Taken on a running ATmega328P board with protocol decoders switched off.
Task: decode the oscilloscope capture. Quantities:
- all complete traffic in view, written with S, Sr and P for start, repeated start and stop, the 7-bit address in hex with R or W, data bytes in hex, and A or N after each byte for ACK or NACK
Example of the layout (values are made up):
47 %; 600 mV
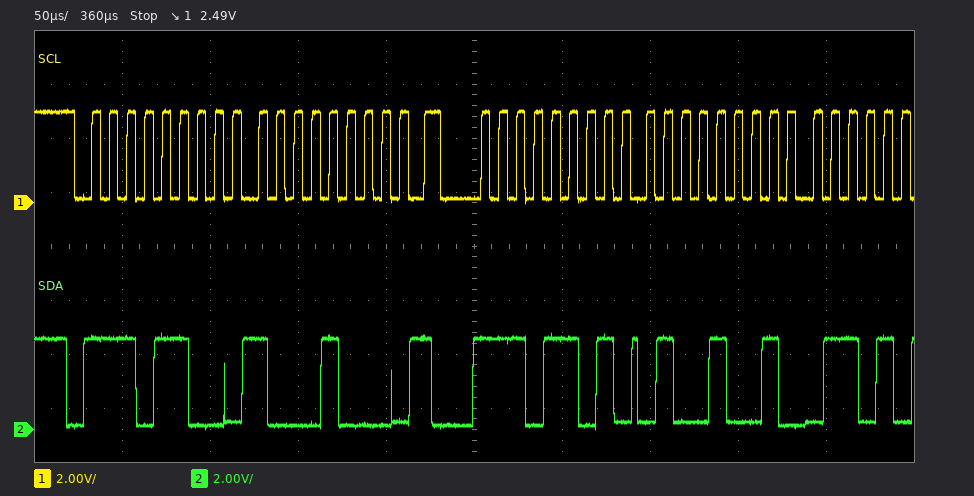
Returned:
S 76W A 88 A Sr 76R A 49 A
